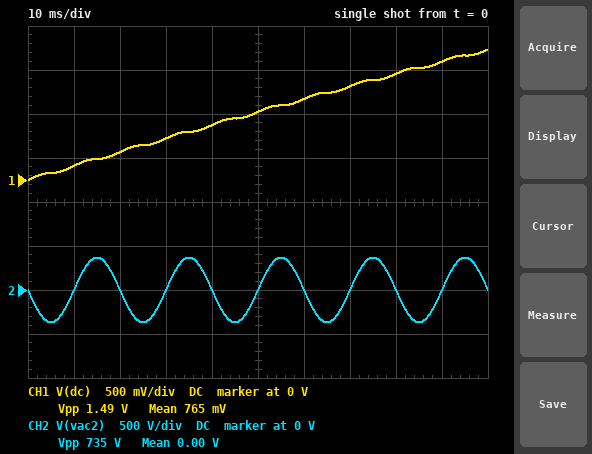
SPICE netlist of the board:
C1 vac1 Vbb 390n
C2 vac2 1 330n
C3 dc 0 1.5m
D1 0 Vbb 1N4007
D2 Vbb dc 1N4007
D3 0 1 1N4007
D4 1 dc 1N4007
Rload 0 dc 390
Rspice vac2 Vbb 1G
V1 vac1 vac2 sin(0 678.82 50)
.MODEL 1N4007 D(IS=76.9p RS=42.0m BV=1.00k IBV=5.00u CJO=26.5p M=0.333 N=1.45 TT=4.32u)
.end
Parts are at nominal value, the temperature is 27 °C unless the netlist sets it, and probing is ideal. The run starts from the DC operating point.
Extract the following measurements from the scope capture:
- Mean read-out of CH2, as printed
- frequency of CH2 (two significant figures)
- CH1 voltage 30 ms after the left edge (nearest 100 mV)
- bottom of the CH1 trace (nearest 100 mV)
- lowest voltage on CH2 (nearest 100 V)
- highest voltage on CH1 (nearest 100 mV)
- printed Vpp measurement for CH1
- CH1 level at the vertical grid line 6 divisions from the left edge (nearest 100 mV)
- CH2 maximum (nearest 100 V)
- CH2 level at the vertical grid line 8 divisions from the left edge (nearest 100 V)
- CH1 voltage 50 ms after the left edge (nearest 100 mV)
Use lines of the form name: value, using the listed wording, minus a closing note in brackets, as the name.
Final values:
Mean read-out of CH2, as printed: 0.00 V
frequency of CH2: 50 Hz
CH1 voltage 30 ms after the left edge: 500 mV
bottom of the CH1 trace: 0 V
lowest voltage on CH2: -400 V
highest voltage on CH1: 1.5 V
printed Vpp measurement for CH1: 1.49 V
CH1 level at the vertical grid line 6 divisions from the left edge: 900 mV
CH2 maximum: 400 V
CH2 level at the vertical grid line 8 divisions from the left edge: 0 V
CH1 voltage 50 ms after the left edge: 800 mV
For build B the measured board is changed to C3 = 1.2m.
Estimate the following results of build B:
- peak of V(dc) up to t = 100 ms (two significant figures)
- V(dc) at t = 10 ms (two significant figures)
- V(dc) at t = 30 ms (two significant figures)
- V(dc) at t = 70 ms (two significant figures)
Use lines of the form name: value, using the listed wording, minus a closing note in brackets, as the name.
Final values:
peak of V(dc) up to t = 100 ms: 1.8 V
V(dc) at t = 10 ms: 200 mV
V(dc) at t = 30 ms: 590 mV
V(dc) at t = 70 ms: 1.3 V
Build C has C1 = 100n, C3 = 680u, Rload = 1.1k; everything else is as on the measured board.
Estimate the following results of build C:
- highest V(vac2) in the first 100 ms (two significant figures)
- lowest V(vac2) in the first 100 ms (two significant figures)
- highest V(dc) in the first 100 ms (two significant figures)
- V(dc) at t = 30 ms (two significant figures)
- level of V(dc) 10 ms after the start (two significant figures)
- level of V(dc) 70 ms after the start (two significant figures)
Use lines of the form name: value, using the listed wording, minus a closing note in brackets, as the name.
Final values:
highest V(vac2) in the first 100 ms: 160 V
lowest V(vac2) in the first 100 ms: -160 V
highest V(dc) in the first 100 ms: 1.4 V
V(dc) at t = 30 ms: 450 mV
level of V(dc) 10 ms after the start: 150 mV
level of V(dc) 70 ms after the start: 1.0 V
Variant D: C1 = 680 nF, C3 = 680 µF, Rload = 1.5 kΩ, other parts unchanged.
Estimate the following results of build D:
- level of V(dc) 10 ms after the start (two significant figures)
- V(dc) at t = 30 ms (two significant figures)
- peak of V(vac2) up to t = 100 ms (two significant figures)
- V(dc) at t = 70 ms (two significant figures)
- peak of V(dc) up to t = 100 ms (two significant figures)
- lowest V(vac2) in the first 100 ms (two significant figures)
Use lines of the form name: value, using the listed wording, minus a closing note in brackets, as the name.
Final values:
level of V(dc) 10 ms after the start: 440 mV
V(dc) at t = 30 ms: 1.3 V
peak of V(vac2) up to t = 100 ms: 460 V
V(dc) at t = 70 ms: 3.0 V
peak of V(dc) up to t = 100 ms: 4.2 V
lowest V(vac2) in the first 100 ms: -460 V
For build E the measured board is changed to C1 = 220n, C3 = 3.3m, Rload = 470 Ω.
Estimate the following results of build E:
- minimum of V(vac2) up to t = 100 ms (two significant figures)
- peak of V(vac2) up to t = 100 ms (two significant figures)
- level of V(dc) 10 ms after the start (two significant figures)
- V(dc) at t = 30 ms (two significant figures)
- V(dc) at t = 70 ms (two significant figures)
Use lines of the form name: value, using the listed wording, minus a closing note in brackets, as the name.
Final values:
minimum of V(vac2) up to t = 100 ms: -270 V
peak of V(vac2) up to t = 100 ms: 270 V
level of V(dc) 10 ms after the start: 54 mV
V(dc) at t = 30 ms: 160 mV
V(dc) at t = 70 ms: 370 mV
